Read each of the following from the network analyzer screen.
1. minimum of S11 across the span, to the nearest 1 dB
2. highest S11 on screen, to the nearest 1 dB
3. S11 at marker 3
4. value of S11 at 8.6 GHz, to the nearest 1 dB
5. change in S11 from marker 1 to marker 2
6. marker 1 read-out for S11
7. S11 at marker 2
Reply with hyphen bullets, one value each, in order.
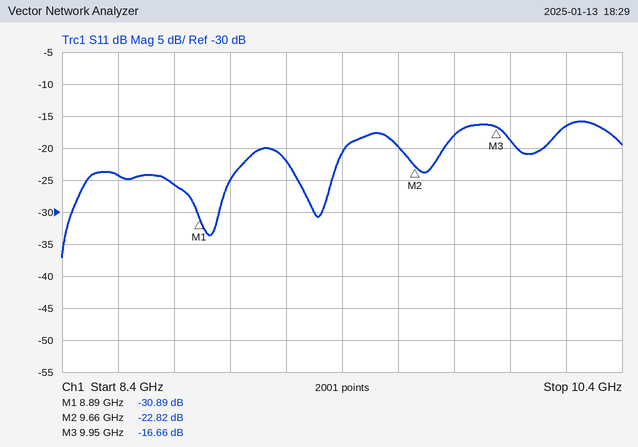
- -37 dB
- -16 dB
- -16.66 dB
- -24 dB
- 8.07 dB
- -30.89 dB
- -22.82 dB
